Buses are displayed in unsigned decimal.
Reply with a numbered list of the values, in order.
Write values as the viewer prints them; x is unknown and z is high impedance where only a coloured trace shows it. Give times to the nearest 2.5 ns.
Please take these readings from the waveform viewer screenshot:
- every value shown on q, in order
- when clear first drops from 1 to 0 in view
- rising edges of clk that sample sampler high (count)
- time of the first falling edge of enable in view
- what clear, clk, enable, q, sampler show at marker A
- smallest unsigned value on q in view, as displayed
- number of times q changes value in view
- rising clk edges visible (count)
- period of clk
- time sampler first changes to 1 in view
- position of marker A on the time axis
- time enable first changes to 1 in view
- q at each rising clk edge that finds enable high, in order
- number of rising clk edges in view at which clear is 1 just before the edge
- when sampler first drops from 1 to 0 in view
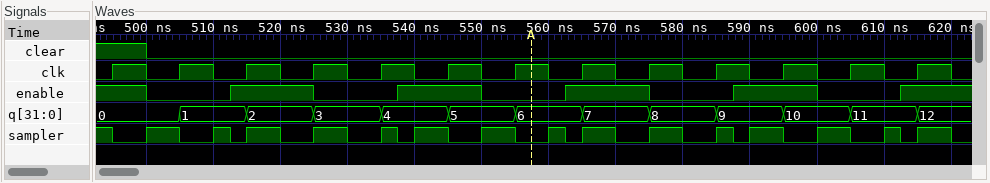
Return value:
1. 0, 1, 2, 3, 4, 5, 6, 7, 8, 9, 10, 11, 12
2. 500 ns
3. 6
4. 500 ns
5. clear=0, clk=1, enable=0, q=6, sampler=0
6. 0
7. 12
8. 13
9. 10 ns
10. 500 ns
11. 557.5 ns
12. 512.5 ns
13. 0, 1, 2, 4, 6, 7, 9, 11
14. 1
15. 495 ns
